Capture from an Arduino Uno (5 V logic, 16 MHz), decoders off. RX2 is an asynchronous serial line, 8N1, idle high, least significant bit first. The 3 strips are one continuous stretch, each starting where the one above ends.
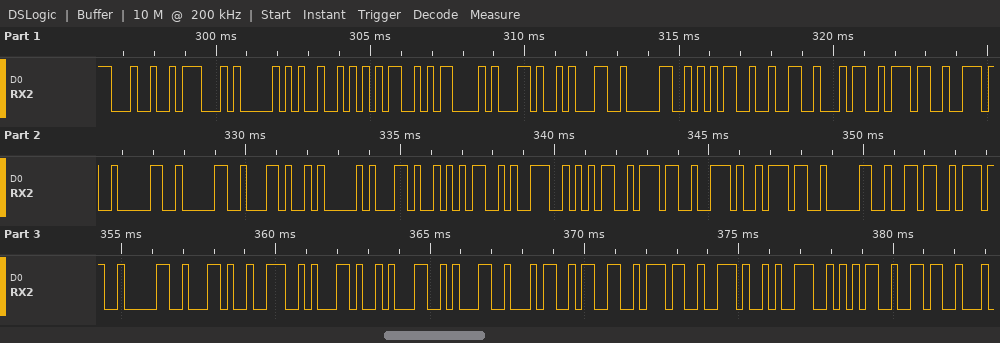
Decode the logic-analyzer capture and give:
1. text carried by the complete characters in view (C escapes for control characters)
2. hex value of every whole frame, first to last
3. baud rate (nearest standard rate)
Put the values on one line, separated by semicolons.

"$GPRMC,105247.00,A,5957.70670,N,11437.956"; 24 47 50 52 4D 43 2C 31 30 35 32 34 37 2E 30 30 2C 41 2C 35 39 35 37 2E 37 30 36 37 30 2C 4E 2C 31 31 34 33 37 2E 39 35 36; 4800 baud
